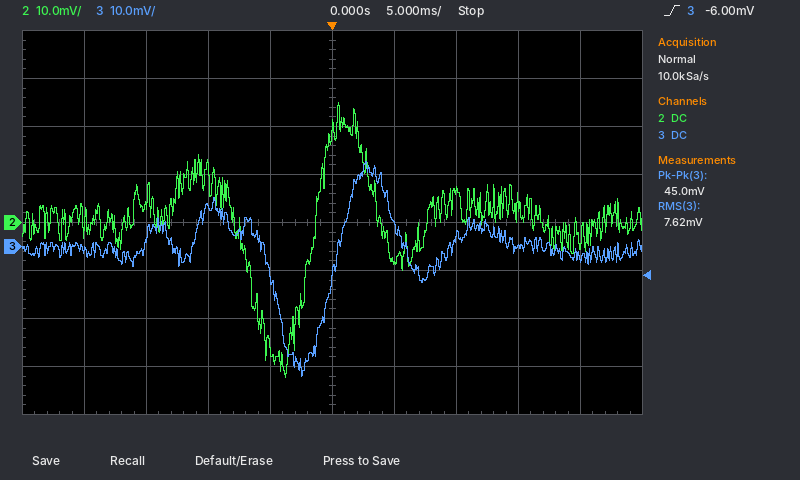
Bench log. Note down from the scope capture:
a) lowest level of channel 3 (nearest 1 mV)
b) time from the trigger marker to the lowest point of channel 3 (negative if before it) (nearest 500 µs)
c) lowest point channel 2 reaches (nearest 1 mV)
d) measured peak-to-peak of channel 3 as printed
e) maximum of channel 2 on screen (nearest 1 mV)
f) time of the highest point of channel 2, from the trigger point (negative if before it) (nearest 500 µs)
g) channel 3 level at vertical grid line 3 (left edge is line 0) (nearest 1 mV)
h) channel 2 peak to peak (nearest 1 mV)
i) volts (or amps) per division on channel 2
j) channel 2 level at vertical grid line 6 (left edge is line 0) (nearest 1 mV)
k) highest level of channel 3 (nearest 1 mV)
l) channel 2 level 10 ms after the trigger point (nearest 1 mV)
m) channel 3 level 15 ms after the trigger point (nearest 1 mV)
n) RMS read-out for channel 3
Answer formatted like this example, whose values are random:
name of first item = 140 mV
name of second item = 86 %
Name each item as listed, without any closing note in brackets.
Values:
lowest level of channel 3 = -27 mV
time from the trigger marker to the lowest point of channel 3 (negative if before it) = -2.5 ms
lowest point channel 2 reaches = -32 mV
measured peak-to-peak of channel 3 as printed = 45.0 mV
maximum of channel 2 on screen = 25 mV
time of the highest point of channel 2, from the trigger point (negative if before it) = +500 µs
channel 3 level at vertical grid line 3 (left edge is line 0) = 8 mV
channel 2 peak to peak = 57 mV
volts (or amps) per division on channel 2 = 10 mV
channel 2 level at vertical grid line 6 (left edge is line 0) = -8 mV
highest level of channel 3 = 18 mV
channel 2 level 10 ms after the trigger point = 7 mV
channel 3 level 15 ms after the trigger point = 0 mV
RMS read-out for channel 3 = 7.62 mV
